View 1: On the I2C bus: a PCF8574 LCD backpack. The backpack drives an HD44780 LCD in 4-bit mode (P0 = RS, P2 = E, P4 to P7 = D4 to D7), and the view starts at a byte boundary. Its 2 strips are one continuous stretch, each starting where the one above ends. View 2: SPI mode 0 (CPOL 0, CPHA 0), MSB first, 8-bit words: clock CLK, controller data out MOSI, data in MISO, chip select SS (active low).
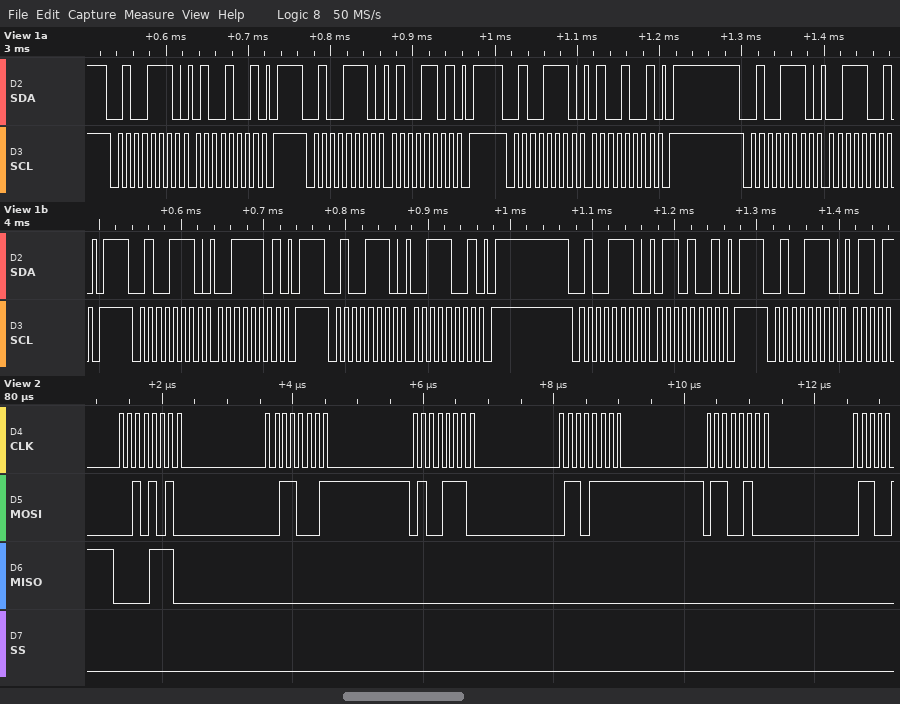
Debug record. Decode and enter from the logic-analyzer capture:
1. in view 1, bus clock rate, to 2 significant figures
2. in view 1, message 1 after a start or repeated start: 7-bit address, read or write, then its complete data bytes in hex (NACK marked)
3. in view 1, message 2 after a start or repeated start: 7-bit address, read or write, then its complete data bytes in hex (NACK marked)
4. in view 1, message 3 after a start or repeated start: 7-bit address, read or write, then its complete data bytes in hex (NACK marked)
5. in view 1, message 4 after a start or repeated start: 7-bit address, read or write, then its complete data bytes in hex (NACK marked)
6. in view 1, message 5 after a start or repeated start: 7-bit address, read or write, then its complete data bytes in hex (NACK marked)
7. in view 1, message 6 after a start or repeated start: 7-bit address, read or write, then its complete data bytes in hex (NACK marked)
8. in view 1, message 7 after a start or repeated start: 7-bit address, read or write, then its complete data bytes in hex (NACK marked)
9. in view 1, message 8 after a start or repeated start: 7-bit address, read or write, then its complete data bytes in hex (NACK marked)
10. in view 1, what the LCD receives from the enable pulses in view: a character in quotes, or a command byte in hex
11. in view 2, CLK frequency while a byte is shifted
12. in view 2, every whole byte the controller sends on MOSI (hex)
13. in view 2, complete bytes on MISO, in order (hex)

100 kHz
0x27 write: 49
0x27 write: 4D
0x27 write: 49
0x27 write: 39
0x27 write: 3D
0x27 write: 39
0x27 write: 69
0x27 write
'C'
8 MHz
2A 31 4E 6F 64
0E 00 00 00 00
